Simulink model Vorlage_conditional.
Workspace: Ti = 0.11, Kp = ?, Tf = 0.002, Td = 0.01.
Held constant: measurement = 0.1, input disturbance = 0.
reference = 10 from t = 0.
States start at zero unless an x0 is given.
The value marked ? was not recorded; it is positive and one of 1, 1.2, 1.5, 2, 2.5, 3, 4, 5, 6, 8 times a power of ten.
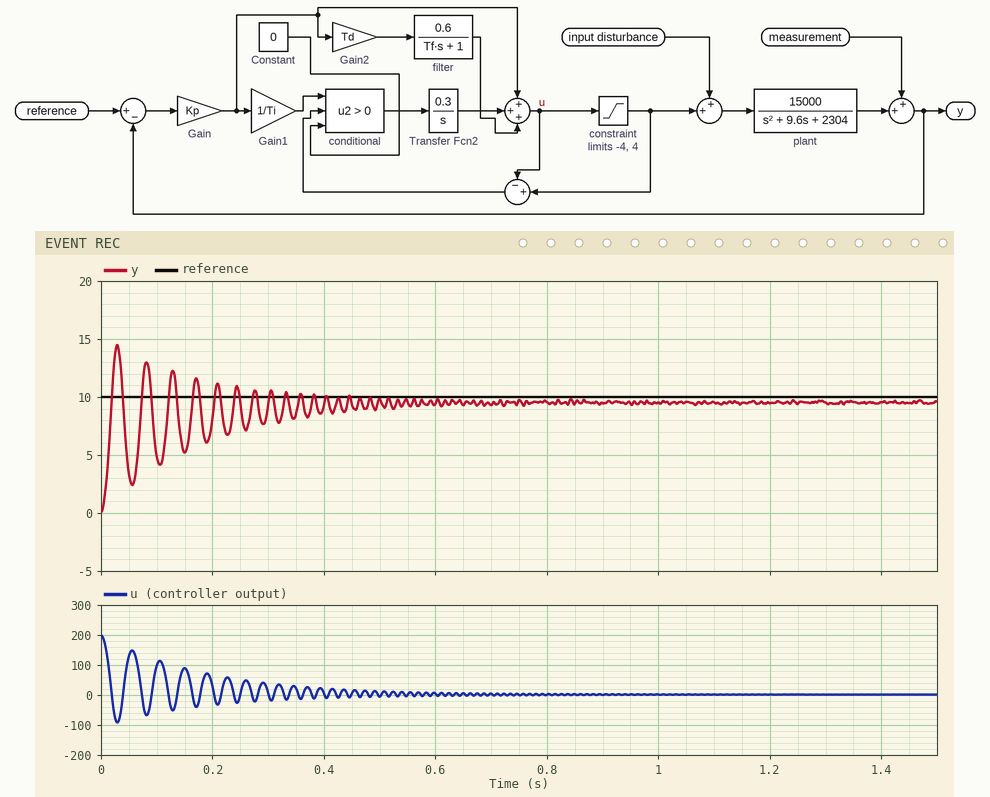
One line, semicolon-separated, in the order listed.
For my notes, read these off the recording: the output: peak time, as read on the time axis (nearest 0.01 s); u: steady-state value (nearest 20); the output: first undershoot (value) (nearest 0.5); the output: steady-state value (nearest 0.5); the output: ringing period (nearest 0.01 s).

0.03 s; 0; 2.5; 9.5; 0.05 s
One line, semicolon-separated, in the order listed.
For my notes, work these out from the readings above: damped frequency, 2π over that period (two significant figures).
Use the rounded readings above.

130 rad/s
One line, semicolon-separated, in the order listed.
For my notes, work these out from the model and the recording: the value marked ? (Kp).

20
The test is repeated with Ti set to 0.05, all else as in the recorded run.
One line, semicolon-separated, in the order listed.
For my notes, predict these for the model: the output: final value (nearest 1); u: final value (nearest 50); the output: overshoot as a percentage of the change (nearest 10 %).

9; 0; 60 %
